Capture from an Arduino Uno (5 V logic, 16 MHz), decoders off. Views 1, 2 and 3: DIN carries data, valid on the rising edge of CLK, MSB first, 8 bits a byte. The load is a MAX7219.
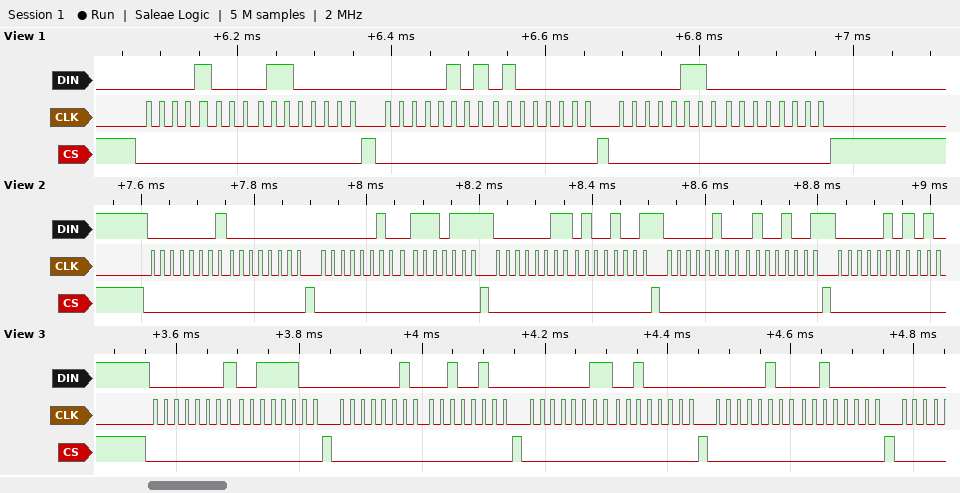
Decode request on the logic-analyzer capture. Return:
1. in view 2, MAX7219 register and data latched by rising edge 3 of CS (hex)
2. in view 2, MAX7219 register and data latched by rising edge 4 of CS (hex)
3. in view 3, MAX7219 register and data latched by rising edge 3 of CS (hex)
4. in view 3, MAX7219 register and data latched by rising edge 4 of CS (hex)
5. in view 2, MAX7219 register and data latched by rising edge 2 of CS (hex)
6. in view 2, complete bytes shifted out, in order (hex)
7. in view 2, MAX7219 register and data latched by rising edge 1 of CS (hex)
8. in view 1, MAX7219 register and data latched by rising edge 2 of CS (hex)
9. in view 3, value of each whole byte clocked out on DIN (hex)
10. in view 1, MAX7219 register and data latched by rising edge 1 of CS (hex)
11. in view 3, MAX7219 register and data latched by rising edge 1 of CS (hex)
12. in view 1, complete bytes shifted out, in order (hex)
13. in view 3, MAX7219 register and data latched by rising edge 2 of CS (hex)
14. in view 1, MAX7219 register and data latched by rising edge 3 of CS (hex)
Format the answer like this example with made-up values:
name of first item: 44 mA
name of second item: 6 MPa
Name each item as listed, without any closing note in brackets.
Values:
in view 2, MAX7219 register and data latched by rising edge 3 of CS: register 0x3, data 0x49
in view 2, MAX7219 register and data latched by rising edge 4 of CS: register 0x4, data 0x49
in view 3, MAX7219 register and data latched by rising edge 3 of CS: register 0x3, data 0x20
in view 3, MAX7219 register and data latched by rising edge 4 of CS: register 0x4, data 0x20
in view 2, MAX7219 register and data latched by rising edge 2 of CS: register 0x2, data 0x77
in view 2, complete bytes shifted out, in order: 01 00 02 77 03 49 04 49 05
in view 2, MAX7219 register and data latched by rising edge 1 of CS: register 0x1, data 0x00
in view 1, MAX7219 register and data latched by rising edge 2 of CS: register 0x5, data 0x40
in view 3, value of each whole byte clocked out on DIN: 0x01 0x3C 0x02 0x24 0x03 0x20 0x04 0x20
in view 1, MAX7219 register and data latched by rising edge 1 of CS: register 0x8, data 0x60
in view 3, MAX7219 register and data latched by rising edge 1 of CS: register 0x1, data 0x3C
in view 1, complete bytes shifted out, in order: 08 60 05 40 06 00
in view 3, MAX7219 register and data latched by rising edge 2 of CS: register 0x2, data 0x24
in view 1, MAX7219 register and data latched by rising edge 3 of CS: register 0x6, data 0x00
